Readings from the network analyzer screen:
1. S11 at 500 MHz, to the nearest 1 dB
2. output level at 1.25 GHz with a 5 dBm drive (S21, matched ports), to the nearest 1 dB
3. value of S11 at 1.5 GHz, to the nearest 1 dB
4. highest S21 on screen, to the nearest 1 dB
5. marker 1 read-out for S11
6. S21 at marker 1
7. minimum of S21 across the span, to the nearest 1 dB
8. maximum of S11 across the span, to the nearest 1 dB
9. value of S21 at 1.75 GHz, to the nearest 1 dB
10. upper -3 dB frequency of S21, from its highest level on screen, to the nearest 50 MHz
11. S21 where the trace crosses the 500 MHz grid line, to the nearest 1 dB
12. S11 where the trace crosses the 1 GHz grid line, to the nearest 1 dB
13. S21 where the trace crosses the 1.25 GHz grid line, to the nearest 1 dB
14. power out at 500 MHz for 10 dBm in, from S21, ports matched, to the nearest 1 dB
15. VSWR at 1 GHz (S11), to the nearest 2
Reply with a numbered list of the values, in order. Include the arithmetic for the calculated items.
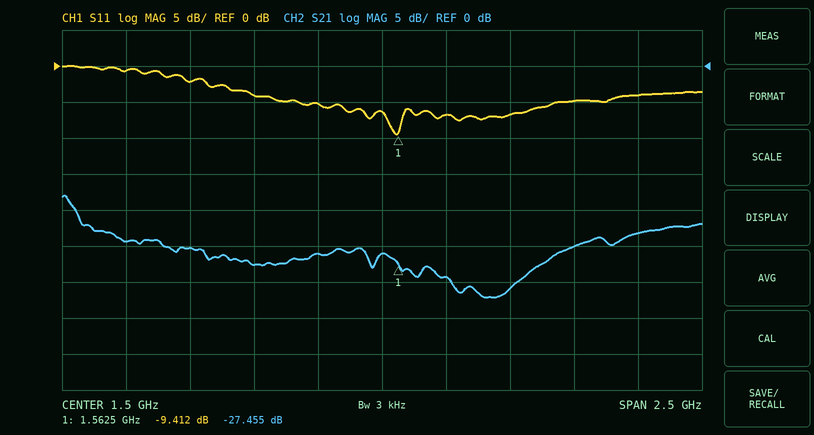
1. -1 dB
2. 5 dBm + (-26 dB) = -21 dBm
3. -6 dB
4. -18 dB
5. -9.412 dB
6. -27.455 dB
7. -32 dB
8. 0 dB
9. -29 dB
10. 300 MHz
11. -24 dB
12. -4 dB
13. -26 dB
14. 10 dBm + (-24 dB) = -14 dBm
15. |Γ| = 10^(-4/20) = 0.6310; VSWR = (1 + 0.6310)/(1 − 0.6310) ≈ 4
